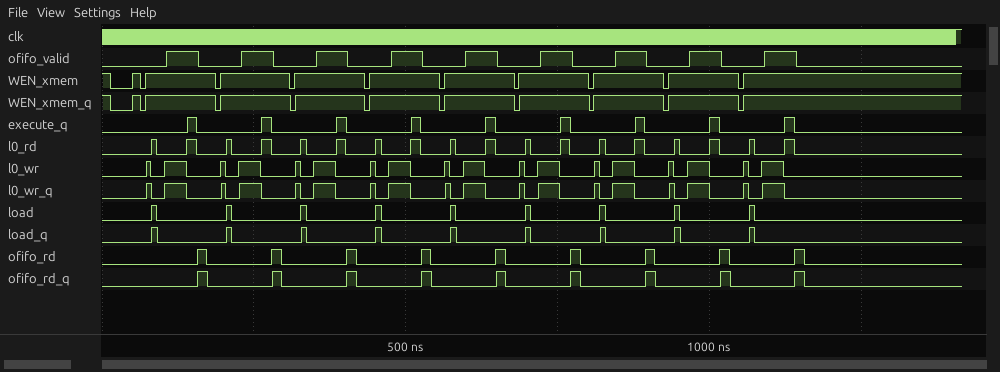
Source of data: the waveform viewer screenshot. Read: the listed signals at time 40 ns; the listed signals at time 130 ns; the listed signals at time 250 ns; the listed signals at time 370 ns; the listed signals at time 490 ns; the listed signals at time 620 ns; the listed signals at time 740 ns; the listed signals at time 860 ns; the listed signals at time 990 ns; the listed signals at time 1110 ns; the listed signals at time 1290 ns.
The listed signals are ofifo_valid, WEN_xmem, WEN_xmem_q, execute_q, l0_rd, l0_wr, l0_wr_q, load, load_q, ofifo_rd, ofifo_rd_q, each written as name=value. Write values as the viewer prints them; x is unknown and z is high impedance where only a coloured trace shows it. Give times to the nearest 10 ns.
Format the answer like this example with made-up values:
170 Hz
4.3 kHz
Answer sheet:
ofifo_valid=0, WEN_xmem=0, WEN_xmem_q=0, execute_q=0, l0_rd=0, l0_wr=0, l0_wr_q=0, load=0, load_q=0, ofifo_rd=0, ofifo_rd_q=0
ofifo_valid=1, WEN_xmem=1, WEN_xmem_q=1, execute_q=0, l0_rd=0, l0_wr=1, l0_wr_q=1, load=0, load_q=0, ofifo_rd=0, ofifo_rd_q=0
ofifo_valid=1, WEN_xmem=1, WEN_xmem_q=1, execute_q=0, l0_rd=0, l0_wr=1, l0_wr_q=1, load=0, load_q=0, ofifo_rd=0, ofifo_rd_q=0
ofifo_valid=1, WEN_xmem=1, WEN_xmem_q=1, execute_q=0, l0_rd=0, l0_wr=1, l0_wr_q=1, load=0, load_q=0, ofifo_rd=0, ofifo_rd_q=0
ofifo_valid=1, WEN_xmem=1, WEN_xmem_q=1, execute_q=0, l0_rd=0, l0_wr=1, l0_wr_q=1, load=0, load_q=0, ofifo_rd=0, ofifo_rd_q=0
ofifo_valid=1, WEN_xmem=1, WEN_xmem_q=1, execute_q=0, l0_rd=0, l0_wr=1, l0_wr_q=1, load=0, load_q=0, ofifo_rd=0, ofifo_rd_q=0
ofifo_valid=1, WEN_xmem=1, WEN_xmem_q=1, execute_q=0, l0_rd=0, l0_wr=1, l0_wr_q=1, load=0, load_q=0, ofifo_rd=0, ofifo_rd_q=0
ofifo_valid=1, WEN_xmem=1, WEN_xmem_q=1, execute_q=0, l0_rd=0, l0_wr=1, l0_wr_q=1, load=0, load_q=0, ofifo_rd=0, ofifo_rd_q=0
ofifo_valid=1, WEN_xmem=1, WEN_xmem_q=1, execute_q=0, l0_rd=0, l0_wr=1, l0_wr_q=1, load=0, load_q=0, ofifo_rd=0, ofifo_rd_q=0
ofifo_valid=1, WEN_xmem=1, WEN_xmem_q=1, execute_q=0, l0_rd=0, l0_wr=1, l0_wr_q=1, load=0, load_q=0, ofifo_rd=0, ofifo_rd_q=0
ofifo_valid=0, WEN_xmem=1, WEN_xmem_q=1, execute_q=0, l0_rd=0, l0_wr=0, l0_wr_q=0, load=0, load_q=0, ofifo_rd=0, ofifo_rd_q=0
